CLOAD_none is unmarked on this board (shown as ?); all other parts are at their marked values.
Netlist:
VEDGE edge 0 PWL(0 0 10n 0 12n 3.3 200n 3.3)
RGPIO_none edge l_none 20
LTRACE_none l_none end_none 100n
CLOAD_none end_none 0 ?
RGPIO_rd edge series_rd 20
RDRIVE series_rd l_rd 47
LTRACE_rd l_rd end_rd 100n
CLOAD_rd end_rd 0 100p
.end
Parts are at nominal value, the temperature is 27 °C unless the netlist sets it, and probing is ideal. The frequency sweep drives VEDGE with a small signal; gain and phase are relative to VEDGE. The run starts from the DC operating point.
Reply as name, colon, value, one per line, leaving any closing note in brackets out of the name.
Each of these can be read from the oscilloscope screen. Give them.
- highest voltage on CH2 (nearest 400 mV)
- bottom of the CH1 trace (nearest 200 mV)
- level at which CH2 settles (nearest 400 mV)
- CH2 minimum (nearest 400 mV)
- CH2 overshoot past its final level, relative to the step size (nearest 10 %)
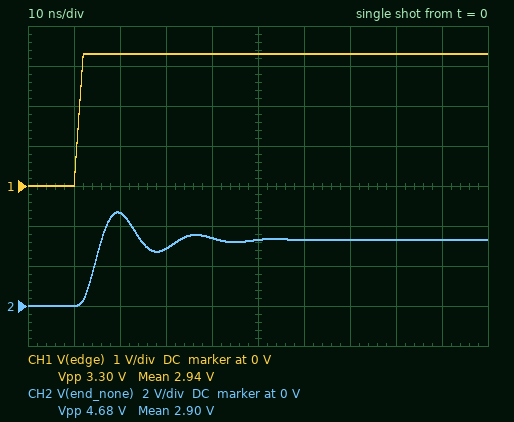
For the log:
highest voltage on CH2: 4.8 V
bottom of the CH1 trace: 0 V
level at which CH2 settles: 3.2 V
CH2 minimum: 0 V
CH2 overshoot past its final level, relative to the step size: 40 %
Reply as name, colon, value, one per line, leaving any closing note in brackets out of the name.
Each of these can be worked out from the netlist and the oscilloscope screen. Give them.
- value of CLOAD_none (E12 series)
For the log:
value of CLOAD_none: 68 pF
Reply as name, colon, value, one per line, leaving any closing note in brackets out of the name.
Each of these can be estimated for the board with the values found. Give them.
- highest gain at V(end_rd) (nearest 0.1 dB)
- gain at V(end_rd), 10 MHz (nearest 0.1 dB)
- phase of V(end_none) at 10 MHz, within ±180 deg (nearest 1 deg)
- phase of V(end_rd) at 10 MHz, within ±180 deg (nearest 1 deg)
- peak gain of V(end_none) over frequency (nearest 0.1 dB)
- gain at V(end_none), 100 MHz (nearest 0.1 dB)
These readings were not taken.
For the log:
highest gain at V(end_rd): 0 dB
gain at V(end_rd), 10 MHz: -0.4 dB
phase of V(end_none) at 10 MHz, within ±180 deg: -5 deg
phase of V(end_rd) at 10 MHz, within ±180 deg: -24 deg
peak gain of V(end_none) over frequency: 6.0 dB
gain at V(end_none), 100 MHz: -5.5 dB
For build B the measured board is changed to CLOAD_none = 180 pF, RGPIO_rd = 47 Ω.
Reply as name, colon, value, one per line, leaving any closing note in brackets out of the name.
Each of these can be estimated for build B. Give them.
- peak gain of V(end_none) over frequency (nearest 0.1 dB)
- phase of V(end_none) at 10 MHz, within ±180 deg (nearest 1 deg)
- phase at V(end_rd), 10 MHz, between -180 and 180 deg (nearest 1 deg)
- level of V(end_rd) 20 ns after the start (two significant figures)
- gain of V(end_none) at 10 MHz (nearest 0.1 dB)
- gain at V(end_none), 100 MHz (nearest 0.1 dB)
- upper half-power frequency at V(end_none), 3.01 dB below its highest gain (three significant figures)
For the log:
peak gain of V(end_none) over frequency: 2.3 dB
phase of V(end_none) at 10 MHz, within ±180 deg: -14 deg
phase at V(end_rd), 10 MHz, between -180 and 180 deg: -32 deg
level of V(end_rd) 20 ns after the start: 2.0 V
gain of V(end_none) at 10 MHz: 0.4 dB
gain at V(end_none), 100 MHz: -16.3 dB
upper half-power frequency at V(end_none), 3.01 dB below its highest gain: 44.5 MHz
